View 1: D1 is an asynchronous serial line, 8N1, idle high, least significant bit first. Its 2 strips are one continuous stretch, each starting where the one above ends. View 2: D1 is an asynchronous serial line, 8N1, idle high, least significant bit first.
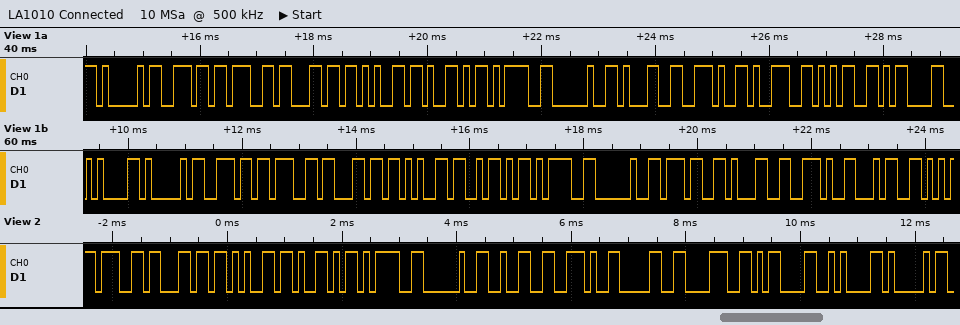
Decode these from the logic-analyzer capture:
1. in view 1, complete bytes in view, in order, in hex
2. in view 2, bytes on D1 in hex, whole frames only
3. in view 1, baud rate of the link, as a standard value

41 6E 67 6C 65 59 3D 20 31 2E 39 35 0D 0A 41 6E 67 6C 65 5A 3D 20 37 31 2E 34
67 6C 65 59 3D 20 32 2E 30 38 0D 0A 41
9600 baud
